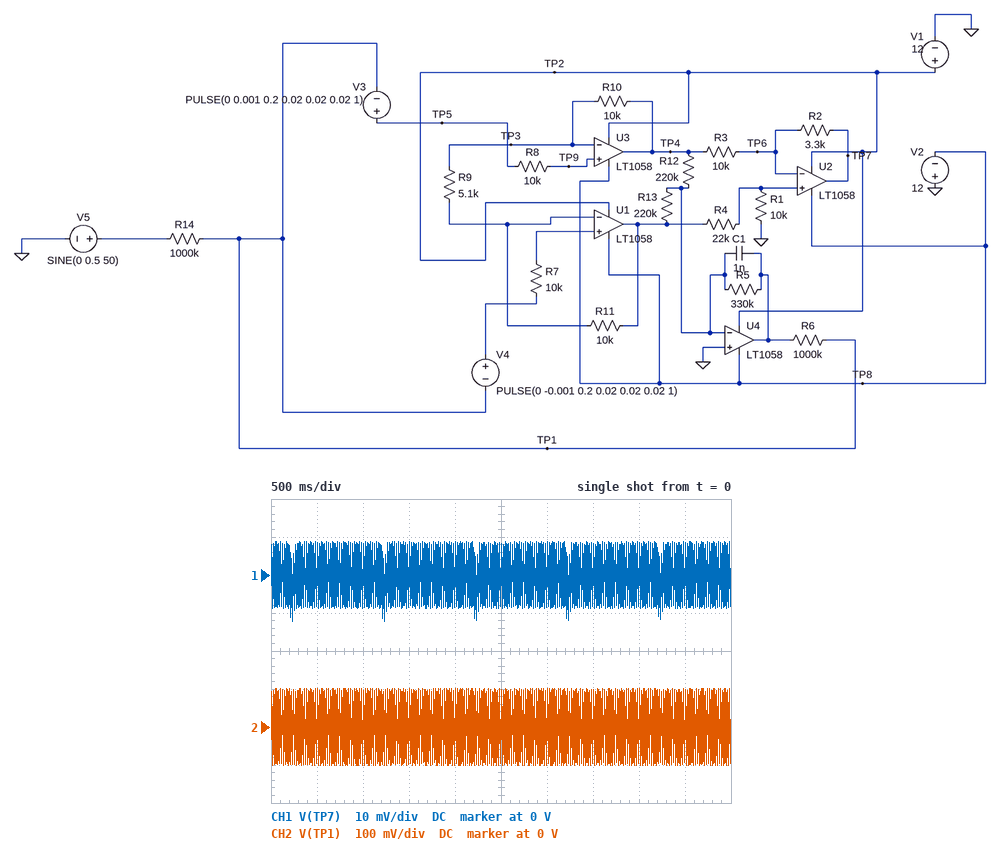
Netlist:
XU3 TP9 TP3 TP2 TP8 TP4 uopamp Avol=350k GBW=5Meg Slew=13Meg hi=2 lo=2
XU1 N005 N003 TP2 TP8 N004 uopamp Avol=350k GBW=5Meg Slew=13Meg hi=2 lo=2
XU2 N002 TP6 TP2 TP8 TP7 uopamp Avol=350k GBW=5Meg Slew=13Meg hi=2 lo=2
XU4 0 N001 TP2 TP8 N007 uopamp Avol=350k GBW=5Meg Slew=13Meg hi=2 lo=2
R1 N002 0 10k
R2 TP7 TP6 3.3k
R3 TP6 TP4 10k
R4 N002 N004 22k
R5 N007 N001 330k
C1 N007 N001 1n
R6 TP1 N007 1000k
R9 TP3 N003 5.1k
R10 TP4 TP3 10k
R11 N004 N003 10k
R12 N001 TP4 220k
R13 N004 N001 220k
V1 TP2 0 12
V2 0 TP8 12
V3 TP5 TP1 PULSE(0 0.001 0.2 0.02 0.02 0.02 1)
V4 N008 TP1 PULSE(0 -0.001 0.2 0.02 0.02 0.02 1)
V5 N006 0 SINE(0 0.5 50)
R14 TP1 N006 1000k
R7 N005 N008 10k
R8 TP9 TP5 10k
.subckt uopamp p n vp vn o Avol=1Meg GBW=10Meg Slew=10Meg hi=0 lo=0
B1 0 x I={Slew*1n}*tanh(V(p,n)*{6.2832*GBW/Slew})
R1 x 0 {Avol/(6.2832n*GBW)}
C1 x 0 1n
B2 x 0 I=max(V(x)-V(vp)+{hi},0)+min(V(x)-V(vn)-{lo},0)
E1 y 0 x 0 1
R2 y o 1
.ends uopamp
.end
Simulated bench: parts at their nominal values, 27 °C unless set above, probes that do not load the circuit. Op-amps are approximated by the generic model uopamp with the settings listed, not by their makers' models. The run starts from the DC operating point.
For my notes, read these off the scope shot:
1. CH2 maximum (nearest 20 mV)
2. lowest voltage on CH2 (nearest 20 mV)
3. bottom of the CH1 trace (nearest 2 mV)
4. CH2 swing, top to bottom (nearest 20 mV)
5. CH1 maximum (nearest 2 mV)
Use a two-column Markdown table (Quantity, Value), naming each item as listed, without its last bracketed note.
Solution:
| Quantity | Value |
|---|---|
| CH2 maximum | 100 mV |
| lowest voltage on CH2 | -100 mV |
| bottom of the CH1 trace | -12 mV |
| CH2 swing, top to bottom | 200 mV |
| CH1 maximum | 8 mV |
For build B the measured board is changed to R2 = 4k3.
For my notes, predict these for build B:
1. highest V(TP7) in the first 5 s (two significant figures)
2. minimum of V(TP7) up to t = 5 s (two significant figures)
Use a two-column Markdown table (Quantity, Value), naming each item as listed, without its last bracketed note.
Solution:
| Quantity | Value |
|---|---|
| highest V(TP7) in the first 5 s | 1.7 mV |
| minimum of V(TP7) up to t = 5 s | -6.0 mV |
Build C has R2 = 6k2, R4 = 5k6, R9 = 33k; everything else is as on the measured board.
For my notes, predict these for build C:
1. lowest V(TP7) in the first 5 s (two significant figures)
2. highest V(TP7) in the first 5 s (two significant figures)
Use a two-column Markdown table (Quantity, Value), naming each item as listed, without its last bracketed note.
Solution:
| Quantity | Value |
|---|---|
| lowest V(TP7) in the first 5 s | -45 mV |
| highest V(TP7) in the first 5 s | 42 mV |
